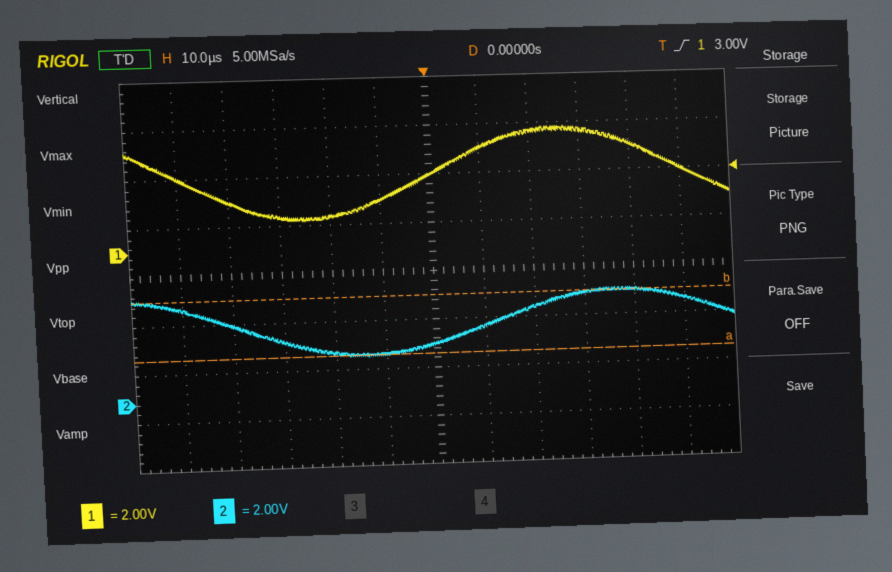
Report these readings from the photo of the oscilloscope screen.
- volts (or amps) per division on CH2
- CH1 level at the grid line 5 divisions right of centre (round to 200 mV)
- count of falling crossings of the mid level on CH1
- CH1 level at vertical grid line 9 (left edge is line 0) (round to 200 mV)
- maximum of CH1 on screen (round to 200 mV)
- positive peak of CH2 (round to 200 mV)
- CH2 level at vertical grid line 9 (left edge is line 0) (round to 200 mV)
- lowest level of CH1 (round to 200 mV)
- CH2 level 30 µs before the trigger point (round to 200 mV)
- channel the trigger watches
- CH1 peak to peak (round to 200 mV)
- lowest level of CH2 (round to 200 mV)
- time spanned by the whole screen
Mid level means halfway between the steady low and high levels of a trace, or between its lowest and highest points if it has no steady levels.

2 V
3.0 V
2
4.6 V
4.8 V
4.2 V
4.2 V
1.2 V
2.4 V
CH1
3.6 V
1.8 V
120 µs
